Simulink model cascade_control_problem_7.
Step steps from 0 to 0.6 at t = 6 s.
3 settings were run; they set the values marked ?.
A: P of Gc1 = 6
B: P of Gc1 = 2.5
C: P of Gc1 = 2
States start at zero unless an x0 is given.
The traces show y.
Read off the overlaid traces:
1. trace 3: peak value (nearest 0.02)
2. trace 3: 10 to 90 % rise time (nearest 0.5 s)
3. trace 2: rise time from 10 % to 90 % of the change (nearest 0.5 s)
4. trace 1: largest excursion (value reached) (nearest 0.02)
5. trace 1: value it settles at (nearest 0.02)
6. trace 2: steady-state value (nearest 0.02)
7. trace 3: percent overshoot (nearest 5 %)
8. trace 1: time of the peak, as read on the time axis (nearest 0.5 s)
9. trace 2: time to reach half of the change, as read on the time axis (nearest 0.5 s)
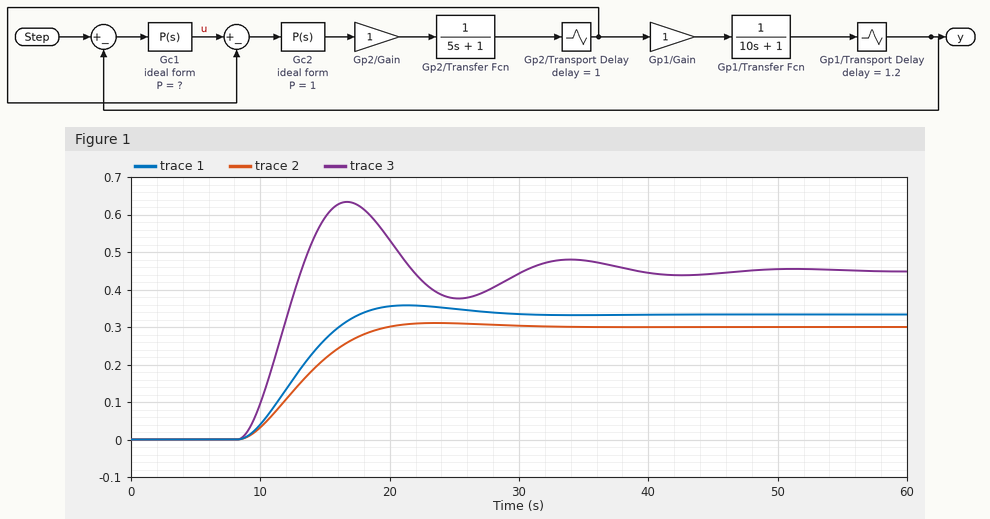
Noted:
0.64
3.5 s
7.5 s
0.36
0.34
0.30
40 %
21.5 s
13.0 s
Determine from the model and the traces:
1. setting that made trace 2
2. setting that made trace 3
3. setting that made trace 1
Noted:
C
A
B
